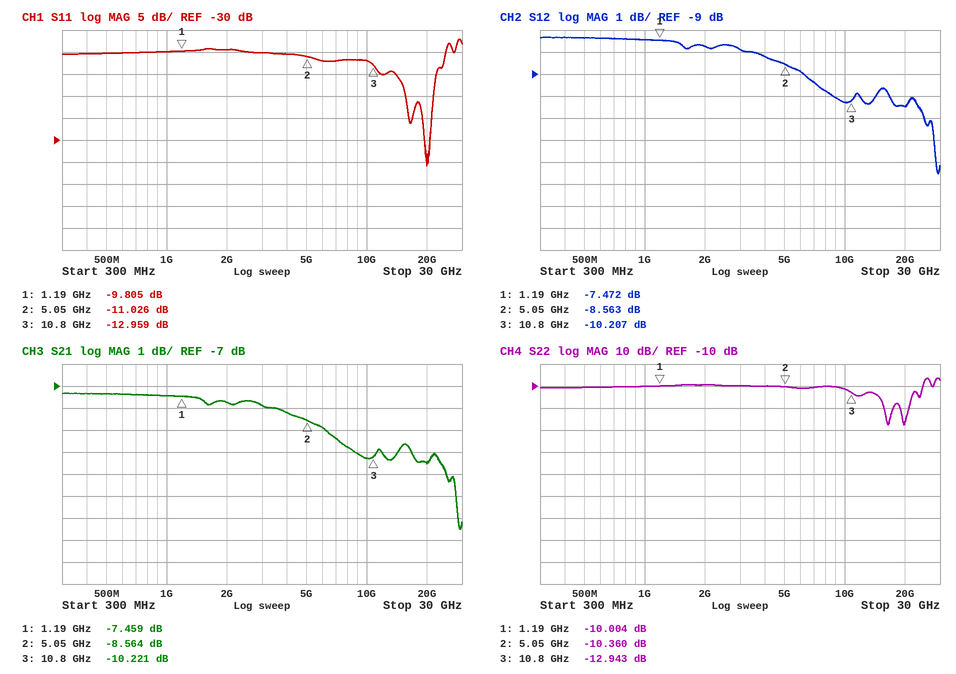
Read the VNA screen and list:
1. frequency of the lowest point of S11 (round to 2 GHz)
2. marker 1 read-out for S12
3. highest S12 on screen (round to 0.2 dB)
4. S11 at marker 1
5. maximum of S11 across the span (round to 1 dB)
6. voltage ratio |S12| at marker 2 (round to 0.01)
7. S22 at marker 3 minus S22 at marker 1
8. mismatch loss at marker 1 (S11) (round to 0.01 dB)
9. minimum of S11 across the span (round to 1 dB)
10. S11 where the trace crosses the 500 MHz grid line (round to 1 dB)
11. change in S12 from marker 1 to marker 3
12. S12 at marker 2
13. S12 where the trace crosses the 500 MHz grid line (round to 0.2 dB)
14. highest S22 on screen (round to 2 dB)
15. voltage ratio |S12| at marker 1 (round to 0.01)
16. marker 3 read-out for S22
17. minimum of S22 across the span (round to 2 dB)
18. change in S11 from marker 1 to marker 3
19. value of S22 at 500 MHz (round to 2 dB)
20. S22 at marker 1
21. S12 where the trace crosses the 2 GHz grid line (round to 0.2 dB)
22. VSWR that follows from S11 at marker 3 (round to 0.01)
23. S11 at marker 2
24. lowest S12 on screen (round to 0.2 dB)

20 GHz
-7.472 dB
-7.4 dB
-9.805 dB
-7 dB
0.37
-2.939 dB
0.48 dB
-36 dB
-10 dB
-2.735 dB
-8.563 dB
-7.4 dB
-6 dB
0.42
-12.943 dB
-28 dB
-3.154 dB
-10 dB
-10.004 dB
-7.8 dB
1.58
-11.026 dB
-13.6 dB
